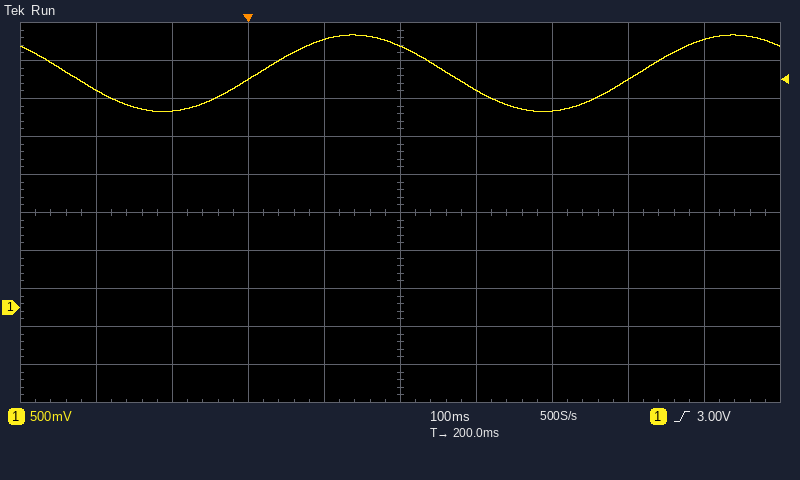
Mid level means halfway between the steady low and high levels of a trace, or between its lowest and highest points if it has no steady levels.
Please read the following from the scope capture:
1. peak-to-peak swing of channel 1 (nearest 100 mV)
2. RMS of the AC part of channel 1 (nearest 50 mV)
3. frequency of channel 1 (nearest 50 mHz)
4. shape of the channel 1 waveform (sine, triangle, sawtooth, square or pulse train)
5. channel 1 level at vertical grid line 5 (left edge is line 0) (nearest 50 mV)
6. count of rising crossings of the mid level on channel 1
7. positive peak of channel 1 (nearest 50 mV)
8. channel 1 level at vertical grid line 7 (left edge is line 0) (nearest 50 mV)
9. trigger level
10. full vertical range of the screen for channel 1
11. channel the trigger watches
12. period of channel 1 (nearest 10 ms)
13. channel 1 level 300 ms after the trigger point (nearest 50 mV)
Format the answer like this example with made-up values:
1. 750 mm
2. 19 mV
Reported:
1. 1.00 V
2. 350 mV
3. 2.00 Hz
4. sine
5. 3.45 V
6. 2
7. 3.60 V
8. 2.60 V
9. 3.00 V
10. 5 V
11. channel 1
12. 500 ms
13. 2.85 V
